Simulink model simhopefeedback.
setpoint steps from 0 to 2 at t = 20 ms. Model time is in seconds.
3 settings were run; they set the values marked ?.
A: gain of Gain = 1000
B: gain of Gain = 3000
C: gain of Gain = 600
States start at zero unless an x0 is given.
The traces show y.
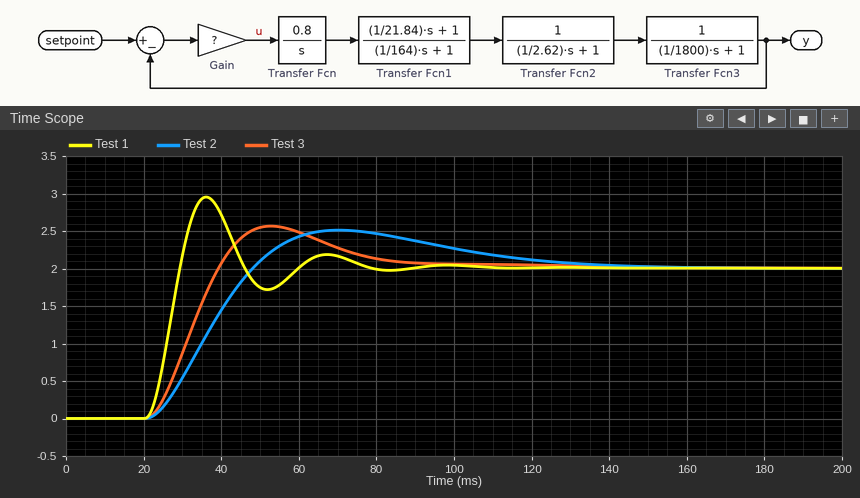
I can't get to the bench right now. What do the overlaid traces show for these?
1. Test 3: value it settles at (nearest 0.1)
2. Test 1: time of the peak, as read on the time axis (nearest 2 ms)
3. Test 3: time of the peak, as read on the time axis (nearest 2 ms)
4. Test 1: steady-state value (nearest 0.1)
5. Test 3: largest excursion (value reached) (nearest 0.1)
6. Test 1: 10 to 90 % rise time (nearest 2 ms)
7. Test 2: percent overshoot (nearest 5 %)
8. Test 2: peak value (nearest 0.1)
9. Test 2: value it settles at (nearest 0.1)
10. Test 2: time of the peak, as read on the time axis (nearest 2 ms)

2.0
36 ms
52 ms
2.0
2.6
6 ms
25 %
2.5
2.0
70 ms
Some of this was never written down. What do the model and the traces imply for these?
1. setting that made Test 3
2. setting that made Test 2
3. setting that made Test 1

A
C
B
